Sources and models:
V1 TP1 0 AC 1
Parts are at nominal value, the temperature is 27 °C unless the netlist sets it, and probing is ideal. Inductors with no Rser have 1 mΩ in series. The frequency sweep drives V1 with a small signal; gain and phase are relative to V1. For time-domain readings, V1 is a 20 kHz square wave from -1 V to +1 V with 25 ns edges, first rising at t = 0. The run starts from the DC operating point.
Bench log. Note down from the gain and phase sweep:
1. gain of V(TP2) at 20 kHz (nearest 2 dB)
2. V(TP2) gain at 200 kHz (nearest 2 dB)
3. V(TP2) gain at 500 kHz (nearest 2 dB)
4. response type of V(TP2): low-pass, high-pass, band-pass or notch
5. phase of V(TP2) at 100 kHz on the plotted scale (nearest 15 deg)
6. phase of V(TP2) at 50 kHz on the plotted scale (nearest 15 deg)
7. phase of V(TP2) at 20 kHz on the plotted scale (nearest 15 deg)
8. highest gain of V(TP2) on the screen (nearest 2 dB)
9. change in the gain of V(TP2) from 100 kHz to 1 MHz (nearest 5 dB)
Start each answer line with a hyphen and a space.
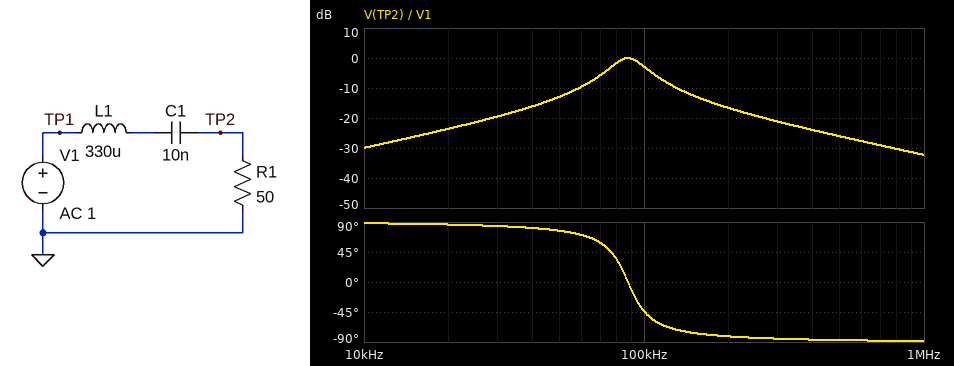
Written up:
- -24 dB
- -16 dB
- -26 dB
- band-pass
- -45 deg
- 75 deg
- 90 deg
- 0 dB
- -30 dB
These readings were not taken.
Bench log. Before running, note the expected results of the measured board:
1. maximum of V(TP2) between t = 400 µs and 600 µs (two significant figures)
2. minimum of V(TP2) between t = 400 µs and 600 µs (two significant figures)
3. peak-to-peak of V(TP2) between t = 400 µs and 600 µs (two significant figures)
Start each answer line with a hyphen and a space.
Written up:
- 410 mV
- -410 mV
- 820 mV
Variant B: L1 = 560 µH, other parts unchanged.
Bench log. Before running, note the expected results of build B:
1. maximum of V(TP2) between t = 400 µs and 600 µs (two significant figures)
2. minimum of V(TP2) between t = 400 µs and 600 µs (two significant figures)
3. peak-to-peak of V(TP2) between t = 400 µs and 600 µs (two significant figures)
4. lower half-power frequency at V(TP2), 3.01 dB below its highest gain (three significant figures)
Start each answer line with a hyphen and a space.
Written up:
- 420 mV
- -420 mV
- 840 mV
- 60.5 kHz
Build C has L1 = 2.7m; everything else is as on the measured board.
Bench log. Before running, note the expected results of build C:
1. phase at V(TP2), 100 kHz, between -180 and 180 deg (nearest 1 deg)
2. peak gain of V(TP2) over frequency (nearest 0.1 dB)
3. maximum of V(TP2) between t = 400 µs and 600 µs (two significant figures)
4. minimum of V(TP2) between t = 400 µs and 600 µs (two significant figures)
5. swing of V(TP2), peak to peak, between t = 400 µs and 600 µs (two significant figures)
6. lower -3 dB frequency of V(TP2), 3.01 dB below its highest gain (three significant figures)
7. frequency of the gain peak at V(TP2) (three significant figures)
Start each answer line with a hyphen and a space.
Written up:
- -88 deg
- 0 dB
- 140 mV
- -140 mV
- 280 mV
- 29.2 kHz
- 30.6 kHz
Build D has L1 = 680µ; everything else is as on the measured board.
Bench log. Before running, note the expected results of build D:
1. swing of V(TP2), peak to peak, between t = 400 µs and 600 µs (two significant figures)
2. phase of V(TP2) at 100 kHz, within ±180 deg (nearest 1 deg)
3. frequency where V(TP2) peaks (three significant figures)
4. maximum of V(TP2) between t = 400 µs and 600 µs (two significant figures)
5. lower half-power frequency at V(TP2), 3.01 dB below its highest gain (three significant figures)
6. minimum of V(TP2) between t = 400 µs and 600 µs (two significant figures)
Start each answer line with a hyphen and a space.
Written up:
- 1.1 V
- -79 deg
- 61.0 kHz
- 550 mV
- 55.5 kHz
- -550 mV
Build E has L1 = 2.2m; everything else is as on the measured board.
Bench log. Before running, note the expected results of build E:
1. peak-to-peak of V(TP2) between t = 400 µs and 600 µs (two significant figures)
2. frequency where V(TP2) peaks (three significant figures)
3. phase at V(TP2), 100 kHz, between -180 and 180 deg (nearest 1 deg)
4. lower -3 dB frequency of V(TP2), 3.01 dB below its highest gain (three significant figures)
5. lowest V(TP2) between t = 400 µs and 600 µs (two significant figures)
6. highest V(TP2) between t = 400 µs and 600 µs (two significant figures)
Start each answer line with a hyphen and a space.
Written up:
- 260 mV
- 33.9 kHz
- -88 deg
- 32.2 kHz
- -130 mV
- 130 mV
